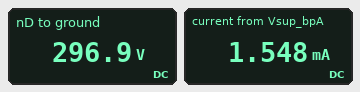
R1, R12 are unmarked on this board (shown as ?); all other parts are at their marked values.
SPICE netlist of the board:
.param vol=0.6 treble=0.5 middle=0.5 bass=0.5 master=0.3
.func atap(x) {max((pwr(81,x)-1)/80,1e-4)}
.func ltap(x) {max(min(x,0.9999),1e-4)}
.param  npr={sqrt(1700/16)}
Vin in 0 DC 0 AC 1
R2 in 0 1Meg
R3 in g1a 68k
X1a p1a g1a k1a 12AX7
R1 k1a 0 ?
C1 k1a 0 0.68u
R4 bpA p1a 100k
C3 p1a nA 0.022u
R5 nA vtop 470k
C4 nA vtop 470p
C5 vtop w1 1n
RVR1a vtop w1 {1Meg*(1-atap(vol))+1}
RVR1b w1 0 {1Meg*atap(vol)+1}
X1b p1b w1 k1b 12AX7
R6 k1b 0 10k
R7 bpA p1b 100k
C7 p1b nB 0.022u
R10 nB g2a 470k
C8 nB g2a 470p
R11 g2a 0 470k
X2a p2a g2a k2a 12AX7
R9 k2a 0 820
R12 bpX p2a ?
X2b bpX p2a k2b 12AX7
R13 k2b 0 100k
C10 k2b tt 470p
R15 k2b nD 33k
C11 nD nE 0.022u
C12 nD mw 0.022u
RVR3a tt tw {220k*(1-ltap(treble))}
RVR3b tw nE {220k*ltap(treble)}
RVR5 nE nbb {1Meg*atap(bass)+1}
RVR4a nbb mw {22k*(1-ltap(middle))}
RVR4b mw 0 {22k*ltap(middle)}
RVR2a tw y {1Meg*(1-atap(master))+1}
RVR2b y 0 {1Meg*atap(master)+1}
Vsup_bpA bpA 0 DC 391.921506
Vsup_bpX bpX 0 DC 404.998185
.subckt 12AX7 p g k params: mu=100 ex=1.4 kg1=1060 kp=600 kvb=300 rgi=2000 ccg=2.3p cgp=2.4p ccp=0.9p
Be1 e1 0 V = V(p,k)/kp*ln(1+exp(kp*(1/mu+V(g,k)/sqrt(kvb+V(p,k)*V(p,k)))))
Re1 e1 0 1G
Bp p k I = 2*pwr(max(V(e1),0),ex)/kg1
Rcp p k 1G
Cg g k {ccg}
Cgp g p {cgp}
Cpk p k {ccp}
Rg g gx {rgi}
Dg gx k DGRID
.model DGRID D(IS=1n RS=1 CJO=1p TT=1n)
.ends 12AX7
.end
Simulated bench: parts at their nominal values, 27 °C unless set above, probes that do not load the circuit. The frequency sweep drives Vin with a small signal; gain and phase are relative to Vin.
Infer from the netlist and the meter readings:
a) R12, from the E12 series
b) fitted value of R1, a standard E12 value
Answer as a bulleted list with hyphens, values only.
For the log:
- 47 kΩ
- 1.8 kΩ
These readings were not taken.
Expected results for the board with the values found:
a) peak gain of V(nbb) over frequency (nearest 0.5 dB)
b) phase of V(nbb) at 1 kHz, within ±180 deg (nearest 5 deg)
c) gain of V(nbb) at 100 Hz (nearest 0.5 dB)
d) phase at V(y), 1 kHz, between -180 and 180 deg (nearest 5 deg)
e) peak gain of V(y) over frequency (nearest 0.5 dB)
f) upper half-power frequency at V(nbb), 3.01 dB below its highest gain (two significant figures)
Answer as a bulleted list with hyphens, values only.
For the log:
- 63.0 dB
- -110 deg
- 35.5 dB
- -105 deg
- 40.5 dB
- 19 kHz
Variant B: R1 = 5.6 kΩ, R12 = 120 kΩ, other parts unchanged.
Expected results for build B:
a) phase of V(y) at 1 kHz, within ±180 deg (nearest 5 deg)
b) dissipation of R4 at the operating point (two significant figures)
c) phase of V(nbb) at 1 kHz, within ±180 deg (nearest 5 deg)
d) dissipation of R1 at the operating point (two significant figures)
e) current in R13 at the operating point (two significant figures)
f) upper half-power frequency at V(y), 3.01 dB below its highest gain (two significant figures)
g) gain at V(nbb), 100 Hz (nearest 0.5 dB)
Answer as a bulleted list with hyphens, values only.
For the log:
- -110 deg
- 33 mW
- -115 deg
- 1.9 mW
- 2.2 mA
- 18 kHz
- 39.5 dB
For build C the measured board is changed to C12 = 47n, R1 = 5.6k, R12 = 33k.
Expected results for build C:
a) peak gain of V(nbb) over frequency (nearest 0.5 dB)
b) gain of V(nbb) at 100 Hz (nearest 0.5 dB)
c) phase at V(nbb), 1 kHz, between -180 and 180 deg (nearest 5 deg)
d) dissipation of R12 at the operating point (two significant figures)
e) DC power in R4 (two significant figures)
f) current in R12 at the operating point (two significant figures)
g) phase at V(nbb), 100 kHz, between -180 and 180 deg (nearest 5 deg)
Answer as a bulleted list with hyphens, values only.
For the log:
- 58.5 dB
- 32.5 dB
- -115 deg
- 220 mW
- 33 mW
- 2.6 mA
- 40 deg
